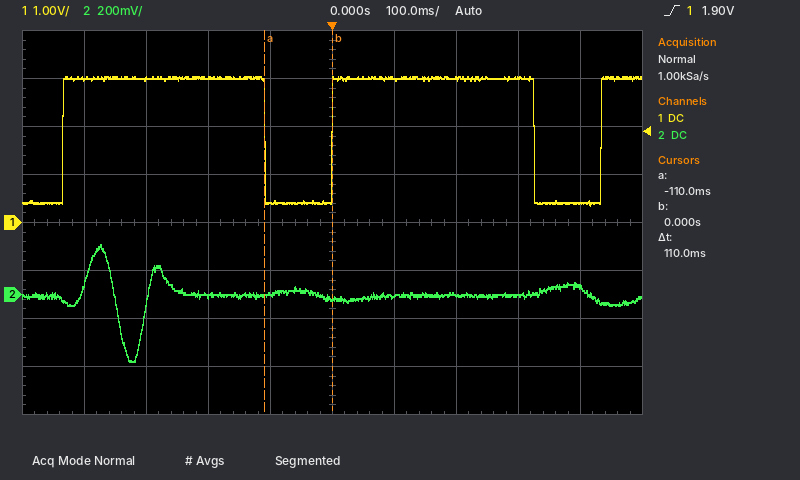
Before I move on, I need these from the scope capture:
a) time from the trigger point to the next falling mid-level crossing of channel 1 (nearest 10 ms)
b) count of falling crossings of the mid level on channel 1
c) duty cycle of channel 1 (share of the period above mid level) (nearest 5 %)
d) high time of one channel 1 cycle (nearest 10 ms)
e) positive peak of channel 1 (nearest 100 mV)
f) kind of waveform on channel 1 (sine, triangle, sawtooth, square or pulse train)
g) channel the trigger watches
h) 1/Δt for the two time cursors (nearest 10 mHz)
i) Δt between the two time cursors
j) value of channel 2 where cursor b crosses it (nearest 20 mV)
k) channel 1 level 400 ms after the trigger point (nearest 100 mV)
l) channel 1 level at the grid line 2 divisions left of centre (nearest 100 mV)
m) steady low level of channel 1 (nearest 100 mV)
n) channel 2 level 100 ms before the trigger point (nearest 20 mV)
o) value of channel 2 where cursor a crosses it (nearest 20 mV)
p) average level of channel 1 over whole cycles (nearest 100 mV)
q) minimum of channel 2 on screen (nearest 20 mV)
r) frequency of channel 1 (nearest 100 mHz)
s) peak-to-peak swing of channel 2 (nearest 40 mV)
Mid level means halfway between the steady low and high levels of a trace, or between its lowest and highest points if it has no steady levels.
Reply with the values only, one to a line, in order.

330 ms
2
75 %
330 ms
3.0 V
pulse train
channel 1
9.09 Hz
110 ms
-20 mV
400 mV
3.0 V
400 mV
0 mV
0 mV
2.4 V
-280 mV
2.3 Hz
480 mV
